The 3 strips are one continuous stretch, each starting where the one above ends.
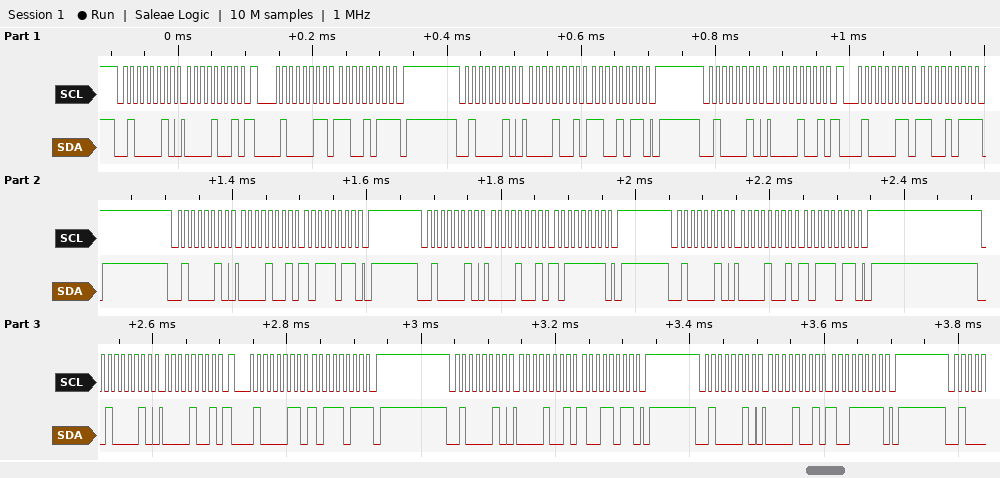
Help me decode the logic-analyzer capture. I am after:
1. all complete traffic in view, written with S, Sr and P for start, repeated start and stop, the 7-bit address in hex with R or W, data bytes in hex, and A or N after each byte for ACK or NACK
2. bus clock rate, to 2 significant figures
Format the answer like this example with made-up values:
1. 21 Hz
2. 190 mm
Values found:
1. S 21W A 09 A Sr 21R A CB N P S 21W A 09 A CB A P S 21W A 09 A Sr 21R A CB N P S 21W A 09 A BB A P S 21W A 09 A BF A P S 21W A 09 A BB A P S 21W A 09 A Sr 21R A BB N P S 21W A 09 A 9B A P S 21W A 09 A 9F A P
2. 100 kHz
